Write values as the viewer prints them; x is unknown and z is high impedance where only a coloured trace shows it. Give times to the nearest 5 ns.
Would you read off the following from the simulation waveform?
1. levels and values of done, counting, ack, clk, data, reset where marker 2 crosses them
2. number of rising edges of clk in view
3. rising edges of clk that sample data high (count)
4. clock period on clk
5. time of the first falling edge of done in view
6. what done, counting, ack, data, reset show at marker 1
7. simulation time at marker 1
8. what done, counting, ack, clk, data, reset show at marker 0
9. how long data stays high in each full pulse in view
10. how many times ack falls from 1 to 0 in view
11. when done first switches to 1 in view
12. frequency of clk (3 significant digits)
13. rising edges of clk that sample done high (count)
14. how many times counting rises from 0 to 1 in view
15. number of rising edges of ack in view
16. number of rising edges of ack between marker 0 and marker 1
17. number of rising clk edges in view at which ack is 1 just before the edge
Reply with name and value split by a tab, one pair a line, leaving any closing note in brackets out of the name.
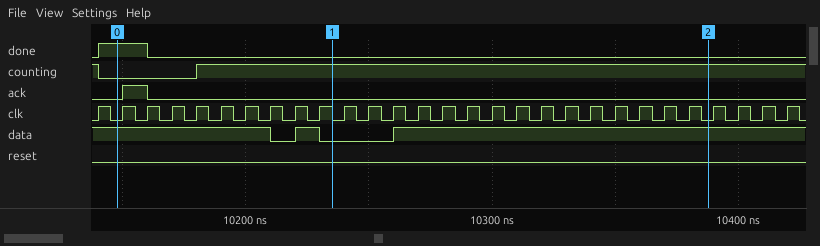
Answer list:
levels and values of done, counting, ack, clk, data, reset where marker 2 crosses them	done=0, counting=1, ack=0, clk=0, data=1, reset=0
number of rising edges of clk in view	29
rising edges of clk that sample data high	25
clock period on clk	10 ns
time of the first falling edge of done in view	10160 ns
what done, counting, ack, data, reset show at marker 1	done=0, counting=1, ack=0, data=0, reset=0
simulation time at marker 1	10235 ns
what done, counting, ack, clk, data, reset show at marker 0	done=1, counting=0, ack=0, clk=0, data=1, reset=0
how long data stays high in each full pulse in view	10 ns
how many times ack falls from 1 to 0 in view	1
when done first switches to 1 in view	10140 ns
frequency of clk	100 MHz
rising edges of clk that sample done high	2
how many times counting rises from 0 to 1 in view	1
number of rising edges of ack in view	1
number of rising edges of ack between marker 0 and marker 1	1
number of rising clk edges in view at which ack is 1 just before the edge	1
